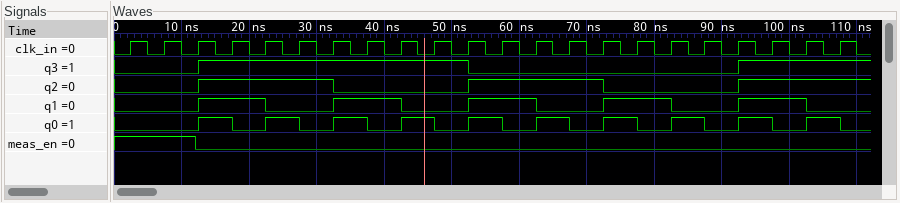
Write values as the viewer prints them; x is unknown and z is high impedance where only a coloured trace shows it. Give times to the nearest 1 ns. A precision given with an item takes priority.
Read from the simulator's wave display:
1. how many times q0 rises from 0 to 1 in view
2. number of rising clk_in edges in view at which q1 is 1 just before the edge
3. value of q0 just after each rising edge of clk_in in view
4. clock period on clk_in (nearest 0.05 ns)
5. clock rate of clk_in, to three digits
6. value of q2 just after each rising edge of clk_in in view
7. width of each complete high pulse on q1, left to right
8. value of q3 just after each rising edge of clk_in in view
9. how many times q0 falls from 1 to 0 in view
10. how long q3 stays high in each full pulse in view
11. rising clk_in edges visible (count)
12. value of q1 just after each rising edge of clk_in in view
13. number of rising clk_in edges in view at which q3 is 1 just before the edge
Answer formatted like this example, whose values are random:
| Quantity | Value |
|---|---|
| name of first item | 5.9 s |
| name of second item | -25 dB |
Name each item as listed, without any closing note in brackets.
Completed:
| Quantity | Value |
|---|---|
| how many times q0 rises from 0 to 1 in view | 10 |
| number of rising clk_in edges in view at which q1 is 1 just before the edge | 10 |
| value of q0 just after each rising edge of clk_in in view | 0 0 1 0 1 0 1 0 1 0 1 0 1 0 1 0 1 0 1 0 1 0 |
| clock period on clk_in | 5 ns |
| clock rate of clk_in, to three digits | 200 MHz |
| value of q2 just after each rising edge of clk_in in view | 0 0 1 1 1 1 0 0 0 0 1 1 1 1 0 0 0 0 1 1 1 1 |
| width of each complete high pulse on q1, left to right | 10 ns, 10 ns, 10 ns, 10 ns, 10 ns |
| value of q3 just after each rising edge of clk_in in view | 0 0 1 1 1 1 1 1 1 1 0 0 0 0 0 0 0 0 1 1 1 1 |
| how many times q0 falls from 1 to 0 in view | 10 |
| how long q3 stays high in each full pulse in view | 40 ns |
| rising clk_in edges visible | 22 |
| value of q1 just after each rising edge of clk_in in view | 0 0 1 1 0 0 1 1 0 0 1 1 0 0 1 1 0 0 1 1 0 0 |
| number of rising clk_in edges in view at which q3 is 1 just before the edge | 11 |
